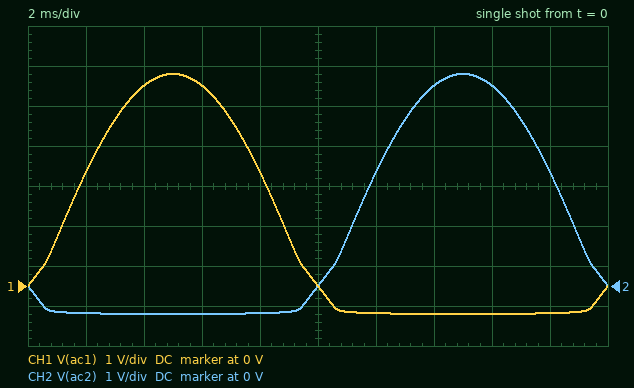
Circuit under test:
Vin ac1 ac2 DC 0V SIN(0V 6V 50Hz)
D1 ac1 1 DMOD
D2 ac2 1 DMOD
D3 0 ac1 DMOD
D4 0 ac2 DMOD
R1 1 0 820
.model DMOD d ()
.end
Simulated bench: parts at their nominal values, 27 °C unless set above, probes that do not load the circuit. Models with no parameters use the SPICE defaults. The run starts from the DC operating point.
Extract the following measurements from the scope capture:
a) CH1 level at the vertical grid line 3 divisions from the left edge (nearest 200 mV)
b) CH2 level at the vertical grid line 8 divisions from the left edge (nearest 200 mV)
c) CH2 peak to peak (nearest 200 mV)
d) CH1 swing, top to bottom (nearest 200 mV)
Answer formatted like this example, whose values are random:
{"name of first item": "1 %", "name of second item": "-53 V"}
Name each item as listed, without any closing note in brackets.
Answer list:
{"CH1 level at the vertical grid line 3 divisions from the left edge": "5.0 V", "CH2 level at the vertical grid line 8 divisions from the left edge": "5.0 V", "CH2 peak to peak": "6.0 V", "CH1 swing, top to bottom": "6.0 V"}
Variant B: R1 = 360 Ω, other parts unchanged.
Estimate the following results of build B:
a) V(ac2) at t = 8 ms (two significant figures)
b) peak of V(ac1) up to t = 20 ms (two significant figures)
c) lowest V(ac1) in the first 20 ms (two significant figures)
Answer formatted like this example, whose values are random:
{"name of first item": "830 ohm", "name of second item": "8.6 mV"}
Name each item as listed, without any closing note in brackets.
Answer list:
{"V(ac2) at t = 8 ms": "-700 mV", "peak of V(ac1) up to t = 20 ms": "5.3 V", "lowest V(ac1) in the first 20 ms": "-720 mV"}
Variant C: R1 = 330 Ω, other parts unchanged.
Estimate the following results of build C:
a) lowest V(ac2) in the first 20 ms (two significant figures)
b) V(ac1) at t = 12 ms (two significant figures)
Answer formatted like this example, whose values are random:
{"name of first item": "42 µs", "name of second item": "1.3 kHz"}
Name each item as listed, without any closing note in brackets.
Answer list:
{"lowest V(ac2) in the first 20 ms": "-720 mV", "V(ac1) at t = 12 ms": "-700 mV"}
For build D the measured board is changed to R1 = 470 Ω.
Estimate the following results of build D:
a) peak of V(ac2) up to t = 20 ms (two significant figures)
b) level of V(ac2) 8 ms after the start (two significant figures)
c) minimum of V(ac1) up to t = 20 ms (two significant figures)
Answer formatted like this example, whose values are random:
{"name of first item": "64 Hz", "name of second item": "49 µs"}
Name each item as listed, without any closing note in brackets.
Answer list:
{"peak of V(ac2) up to t = 20 ms": "5.3 V", "level of V(ac2) 8 ms after the start": "-690 mV", "minimum of V(ac1) up to t = 20 ms": "-710 mV"}
